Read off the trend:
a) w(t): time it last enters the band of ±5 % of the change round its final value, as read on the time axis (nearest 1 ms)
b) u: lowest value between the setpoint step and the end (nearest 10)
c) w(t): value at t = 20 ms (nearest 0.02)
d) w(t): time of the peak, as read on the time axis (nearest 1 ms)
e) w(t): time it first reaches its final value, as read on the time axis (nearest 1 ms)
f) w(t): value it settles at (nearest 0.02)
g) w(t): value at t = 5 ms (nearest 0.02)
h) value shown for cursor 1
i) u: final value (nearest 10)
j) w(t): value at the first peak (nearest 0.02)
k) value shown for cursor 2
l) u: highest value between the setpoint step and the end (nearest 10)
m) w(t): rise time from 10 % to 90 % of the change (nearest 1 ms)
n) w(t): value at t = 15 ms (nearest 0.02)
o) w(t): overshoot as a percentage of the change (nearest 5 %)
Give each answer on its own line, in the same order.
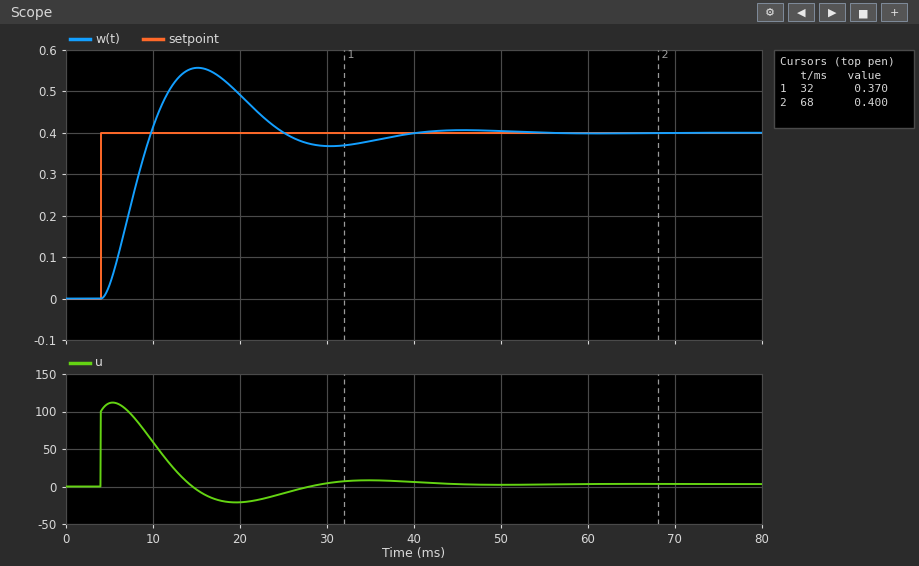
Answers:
35 ms
-20
0.50
15 ms
10 ms
0.40
0.04
0.370
0
0.56
0.400
110
4 ms
0.56
40 %
